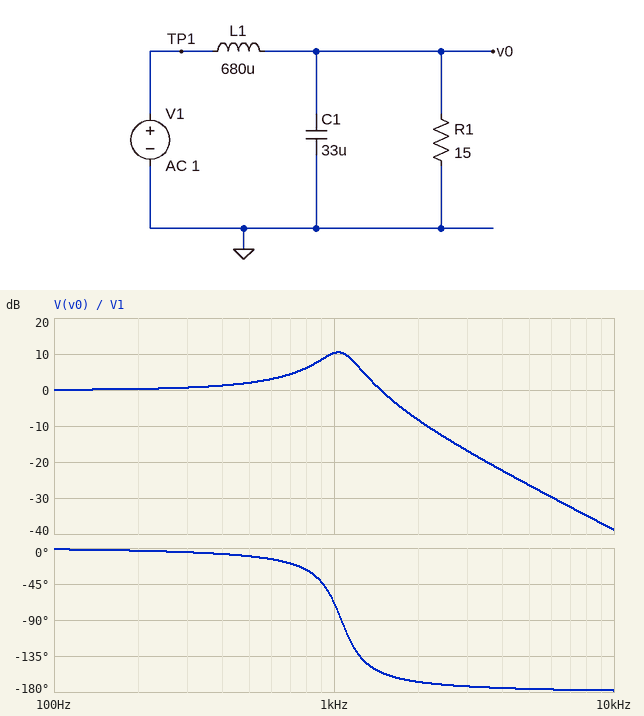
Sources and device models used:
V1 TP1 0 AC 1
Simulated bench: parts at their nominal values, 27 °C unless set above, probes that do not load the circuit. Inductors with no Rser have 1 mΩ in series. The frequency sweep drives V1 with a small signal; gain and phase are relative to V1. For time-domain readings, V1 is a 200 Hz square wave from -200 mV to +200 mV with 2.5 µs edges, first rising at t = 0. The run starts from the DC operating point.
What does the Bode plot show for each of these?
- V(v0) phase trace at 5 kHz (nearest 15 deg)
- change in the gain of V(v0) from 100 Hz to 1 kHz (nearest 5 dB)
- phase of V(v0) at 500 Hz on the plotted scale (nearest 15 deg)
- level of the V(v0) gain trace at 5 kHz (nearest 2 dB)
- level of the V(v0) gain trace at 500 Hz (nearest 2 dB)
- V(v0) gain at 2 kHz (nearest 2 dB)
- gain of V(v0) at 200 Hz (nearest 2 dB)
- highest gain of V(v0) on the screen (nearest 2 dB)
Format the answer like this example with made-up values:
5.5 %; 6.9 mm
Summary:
-180 deg; 10 dB; -15 deg; -26 dB; 2 dB; -8 dB; 0 dB; 10 dB
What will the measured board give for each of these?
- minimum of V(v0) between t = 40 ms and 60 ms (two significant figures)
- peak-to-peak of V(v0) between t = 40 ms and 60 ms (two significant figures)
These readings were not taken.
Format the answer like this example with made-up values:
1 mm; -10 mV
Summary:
-460 mV; 930 mV
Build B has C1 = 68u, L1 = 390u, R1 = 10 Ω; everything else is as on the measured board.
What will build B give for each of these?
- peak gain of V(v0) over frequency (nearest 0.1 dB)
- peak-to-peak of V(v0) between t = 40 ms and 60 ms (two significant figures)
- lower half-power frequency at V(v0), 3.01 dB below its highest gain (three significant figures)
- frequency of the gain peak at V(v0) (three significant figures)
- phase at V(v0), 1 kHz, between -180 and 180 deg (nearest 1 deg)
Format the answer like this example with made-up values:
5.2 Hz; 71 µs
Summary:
12.5 dB; 1.0 V; 837 Hz; 963 Hz; -101 deg
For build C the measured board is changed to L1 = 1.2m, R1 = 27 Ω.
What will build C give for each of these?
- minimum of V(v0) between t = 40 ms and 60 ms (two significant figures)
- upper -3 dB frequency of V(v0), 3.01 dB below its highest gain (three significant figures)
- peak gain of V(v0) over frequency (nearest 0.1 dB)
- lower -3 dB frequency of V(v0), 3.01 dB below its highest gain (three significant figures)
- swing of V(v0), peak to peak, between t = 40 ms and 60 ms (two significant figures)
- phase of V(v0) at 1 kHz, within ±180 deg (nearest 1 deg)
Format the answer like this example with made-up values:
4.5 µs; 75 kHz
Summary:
-430 mV; 875 Hz; 13.1 dB; 694 Hz; 850 mV; -154 deg
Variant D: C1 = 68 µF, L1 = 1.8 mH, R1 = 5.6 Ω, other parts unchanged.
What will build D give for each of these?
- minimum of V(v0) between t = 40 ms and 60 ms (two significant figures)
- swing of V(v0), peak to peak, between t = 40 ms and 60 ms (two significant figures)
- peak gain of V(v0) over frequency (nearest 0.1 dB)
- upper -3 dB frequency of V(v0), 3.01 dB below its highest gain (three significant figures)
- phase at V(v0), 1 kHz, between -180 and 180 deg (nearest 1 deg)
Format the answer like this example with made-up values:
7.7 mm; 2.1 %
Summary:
-280 mV; 550 mV; 1.8 dB; 537 Hz; -152 deg
